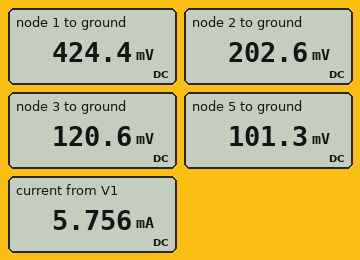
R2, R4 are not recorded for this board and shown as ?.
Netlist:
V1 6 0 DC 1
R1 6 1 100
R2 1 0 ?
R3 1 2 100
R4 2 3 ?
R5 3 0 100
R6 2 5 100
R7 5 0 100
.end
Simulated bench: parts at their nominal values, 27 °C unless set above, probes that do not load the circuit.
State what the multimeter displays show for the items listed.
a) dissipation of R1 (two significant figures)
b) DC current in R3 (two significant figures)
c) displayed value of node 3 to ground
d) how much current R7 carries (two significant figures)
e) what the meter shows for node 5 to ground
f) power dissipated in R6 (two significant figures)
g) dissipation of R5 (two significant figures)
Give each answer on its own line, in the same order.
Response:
3.3 mW
2.2 mA
120.6 mV
1.0 mA
101.3 mV
100 µW
150 µW
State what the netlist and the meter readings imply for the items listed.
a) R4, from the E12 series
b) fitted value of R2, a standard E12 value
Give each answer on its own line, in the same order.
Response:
68 Ω
120 Ω
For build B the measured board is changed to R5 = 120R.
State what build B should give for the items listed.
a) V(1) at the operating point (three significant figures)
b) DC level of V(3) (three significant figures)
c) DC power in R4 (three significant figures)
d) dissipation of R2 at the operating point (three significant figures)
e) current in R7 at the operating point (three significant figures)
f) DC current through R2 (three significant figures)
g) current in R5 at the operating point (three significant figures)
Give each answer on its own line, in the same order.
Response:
427 mV
134 mV
85.0 µW
1.52 mW
1.05 mA
3.56 mA
1.12 mA
